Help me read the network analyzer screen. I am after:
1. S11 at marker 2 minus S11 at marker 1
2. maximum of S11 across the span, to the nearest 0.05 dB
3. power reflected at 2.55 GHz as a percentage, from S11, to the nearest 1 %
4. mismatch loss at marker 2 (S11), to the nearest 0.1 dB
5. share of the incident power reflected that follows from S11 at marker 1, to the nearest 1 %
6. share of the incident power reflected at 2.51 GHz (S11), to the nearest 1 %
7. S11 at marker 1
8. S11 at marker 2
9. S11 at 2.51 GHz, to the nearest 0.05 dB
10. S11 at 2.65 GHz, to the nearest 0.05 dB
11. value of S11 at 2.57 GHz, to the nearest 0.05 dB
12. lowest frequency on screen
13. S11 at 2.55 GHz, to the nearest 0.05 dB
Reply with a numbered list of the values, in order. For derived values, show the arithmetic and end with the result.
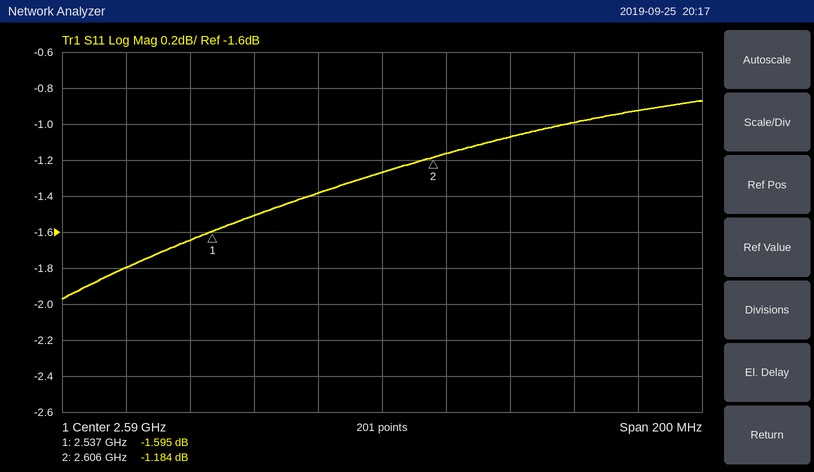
1. -1.184 − (-1.595) = 0.411 dB
2. -0.85 dB
3. 10^(-1.5/10) ≈ 71 %
4. −10 log10(1 − 10^(-1.184/10)) ≈ 6.2 dB
5. 10^(-1.595/10) ≈ 69 %
6. 10^(-1.8/10) ≈ 66 %
7. -1.595 dB
8. -1.184 dB
9. -1.80 dB
10. -1.00 dB
11. -1.40 dB
12. 2.49 GHz
13. -1.50 dB
